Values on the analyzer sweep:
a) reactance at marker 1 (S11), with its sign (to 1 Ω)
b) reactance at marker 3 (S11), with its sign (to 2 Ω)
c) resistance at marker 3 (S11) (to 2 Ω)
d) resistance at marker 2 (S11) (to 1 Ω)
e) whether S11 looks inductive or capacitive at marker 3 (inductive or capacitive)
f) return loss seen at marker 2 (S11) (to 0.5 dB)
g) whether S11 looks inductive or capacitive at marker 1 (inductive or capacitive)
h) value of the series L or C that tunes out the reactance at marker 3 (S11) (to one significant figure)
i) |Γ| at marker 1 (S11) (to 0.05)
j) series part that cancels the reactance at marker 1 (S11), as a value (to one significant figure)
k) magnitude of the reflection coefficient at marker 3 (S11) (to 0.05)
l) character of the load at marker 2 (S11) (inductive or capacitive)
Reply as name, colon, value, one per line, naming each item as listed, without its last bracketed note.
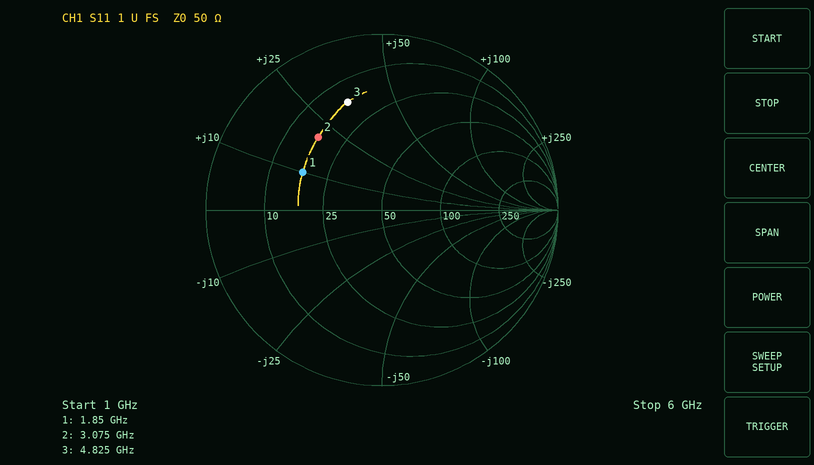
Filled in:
reactance at marker 1 (S11), with its sign: +10 Ω
reactance at marker 3 (S11), with its sign: +34 Ω
resistance at marker 3 (S11): 16 Ω
resistance at marker 2 (S11): 17 Ω
whether S11 looks inductive or capacitive at marker 3: inductive
return loss seen at marker 2 (S11): 5.0 dB
whether S11 looks inductive or capacitive at marker 1: inductive
value of the series L or C that tunes out the reactance at marker 3 (S11): 1.0 pF
|Γ| at marker 1 (S11): 0.50
series part that cancels the reactance at marker 1 (S11), as a value: 9 pF
magnitude of the reflection coefficient at marker 3 (S11): 0.65
character of the load at marker 2 (S11): inductive
